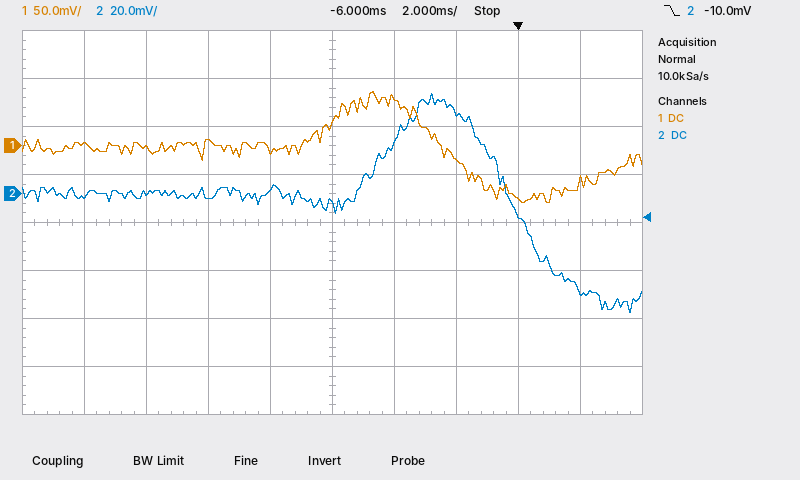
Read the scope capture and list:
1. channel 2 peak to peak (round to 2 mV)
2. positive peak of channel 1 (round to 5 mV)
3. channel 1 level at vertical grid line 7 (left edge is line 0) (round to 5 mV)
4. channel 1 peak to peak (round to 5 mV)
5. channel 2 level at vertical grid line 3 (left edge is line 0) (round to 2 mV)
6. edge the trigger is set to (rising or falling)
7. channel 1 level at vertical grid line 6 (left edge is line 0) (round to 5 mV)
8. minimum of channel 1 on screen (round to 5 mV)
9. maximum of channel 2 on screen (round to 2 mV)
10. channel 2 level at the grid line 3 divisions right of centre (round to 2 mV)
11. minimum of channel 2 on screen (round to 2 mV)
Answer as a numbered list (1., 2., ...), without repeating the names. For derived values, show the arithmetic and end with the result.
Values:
1. 42 mV − (-50 mV) = 92 mV
2. 55 mV
3. -15 mV
4. 55 mV − (-60 mV) = 115 mV
5. -2 mV
6. falling
7. 50 mV
8. -60 mV
9. 42 mV
10. -8 mV
11. -50 mV
